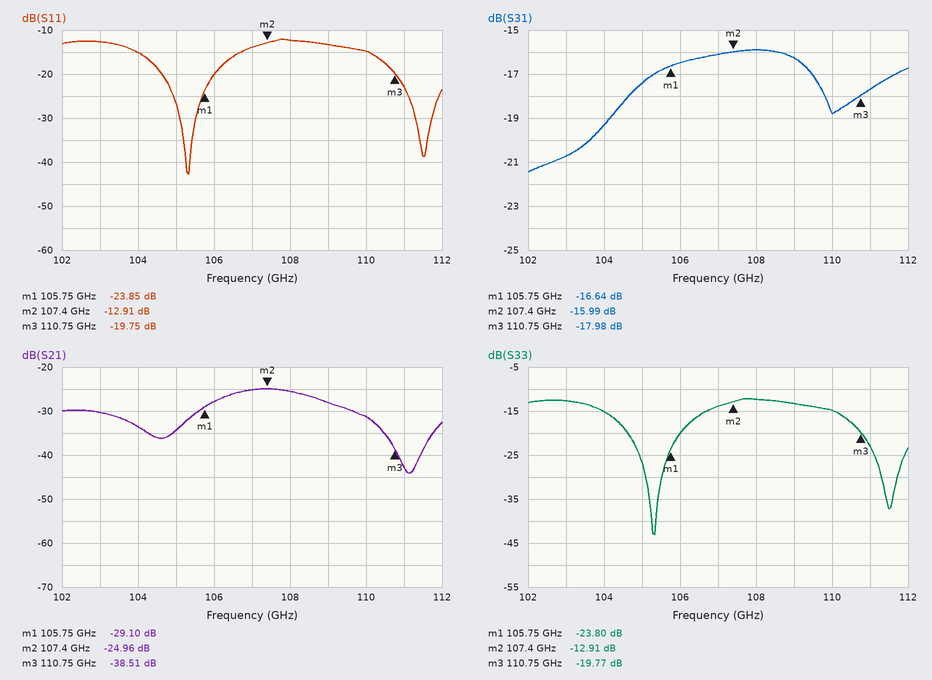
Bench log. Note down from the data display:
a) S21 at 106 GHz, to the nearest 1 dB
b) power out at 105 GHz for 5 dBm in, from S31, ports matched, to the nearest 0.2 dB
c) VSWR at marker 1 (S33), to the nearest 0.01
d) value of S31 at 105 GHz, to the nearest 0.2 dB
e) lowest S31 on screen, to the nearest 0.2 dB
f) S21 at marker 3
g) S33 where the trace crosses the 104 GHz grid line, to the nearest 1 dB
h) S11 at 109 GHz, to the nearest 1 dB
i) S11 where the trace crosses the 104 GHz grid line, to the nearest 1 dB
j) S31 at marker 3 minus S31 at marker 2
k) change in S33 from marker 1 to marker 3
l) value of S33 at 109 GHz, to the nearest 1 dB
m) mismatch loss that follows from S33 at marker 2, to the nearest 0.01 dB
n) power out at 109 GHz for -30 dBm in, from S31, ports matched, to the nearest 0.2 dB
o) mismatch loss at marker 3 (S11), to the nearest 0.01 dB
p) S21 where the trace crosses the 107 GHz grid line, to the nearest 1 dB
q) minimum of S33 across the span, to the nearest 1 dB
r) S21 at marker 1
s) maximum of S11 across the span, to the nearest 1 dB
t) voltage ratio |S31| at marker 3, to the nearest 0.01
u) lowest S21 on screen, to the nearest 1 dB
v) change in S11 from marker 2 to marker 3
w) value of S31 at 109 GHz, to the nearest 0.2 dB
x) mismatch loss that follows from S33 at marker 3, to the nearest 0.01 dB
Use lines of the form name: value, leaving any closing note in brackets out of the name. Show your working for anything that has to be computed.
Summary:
S21 at 106 GHz, to the nearest 1 dB: -28 dB
power out at 105 GHz for 5 dBm in, from S31, ports matched, to the nearest 0.2 dB: 5 dBm + (-17.4 dB) = -12.4 dBm
VSWR at marker 1 (S33), to the nearest 0.01: (1 + 0.0646)/(1 − 0.0646) ≈ 1.14
value of S31 at 105 GHz, to the nearest 0.2 dB: -17.4 dB
lowest S31 on screen, to the nearest 0.2 dB: -21.4 dB
S21 at marker 3: -38.51 dB
S33 where the trace crosses the 104 GHz grid line, to the nearest 1 dB: -15 dB
S11 at 109 GHz, to the nearest 1 dB: -13 dB
S11 where the trace crosses the 104 GHz grid line, to the nearest 1 dB: -15 dB
S31 at marker 3 minus S31 at marker 2: -17.98 − (-15.99) = -1.99 dB
change in S33 from marker 1 to marker 3: -19.77 − (-23.8) = 4.03 dB
value of S33 at 109 GHz, to the nearest 1 dB: -13 dB
mismatch loss that follows from S33 at marker 2, to the nearest 0.01 dB: −10 log10(1 − 10^(-12.91/10)) ≈ 0.23 dB
power out at 109 GHz for -30 dBm in, from S31, ports matched, to the nearest 0.2 dB: -30 dBm + (-16.2 dB) = -46.2 dBm
mismatch loss at marker 3 (S11), to the nearest 0.01 dB: −10 log10(1 − 10^(-19.75/10)) ≈ 0.05 dB
S21 where the trace crosses the 107 GHz grid line, to the nearest 1 dB: -25 dB
minimum of S33 across the span, to the nearest 1 dB: -43 dB
S21 at marker 1: -29.10 dB
maximum of S11 across the span, to the nearest 1 dB: -12 dB
voltage ratio |S31| at marker 3, to the nearest 0.01: 10^(-17.98/20) ≈ 0.13
lowest S21 on screen, to the nearest 1 dB: -44 dB
change in S11 from marker 2 to marker 3: -19.75 − (-12.91) = -6.84 dB
value of S31 at 109 GHz, to the nearest 0.2 dB: -16.2 dB
mismatch loss that follows from S33 at marker 3, to the nearest 0.01 dB: −10 log10(1 − 10^(-19.77/10)) ≈ 0.05 dB
